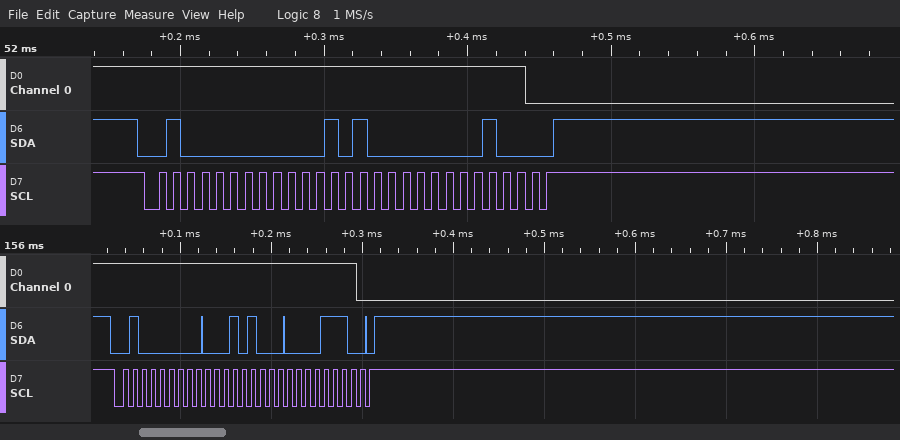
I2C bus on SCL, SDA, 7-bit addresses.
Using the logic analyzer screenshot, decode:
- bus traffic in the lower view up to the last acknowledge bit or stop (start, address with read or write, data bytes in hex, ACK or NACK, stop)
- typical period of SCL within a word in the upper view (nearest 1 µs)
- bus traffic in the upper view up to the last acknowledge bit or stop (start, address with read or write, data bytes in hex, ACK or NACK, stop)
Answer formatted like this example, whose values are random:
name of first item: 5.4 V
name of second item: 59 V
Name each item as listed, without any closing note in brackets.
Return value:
bus traffic in the lower view up to the last acknowledge bit or stop: start, address 20 write ACK, 14 ACK, 0E ACK, stop
typical period of SCL within a word in the upper view: 10 µs
bus traffic in the upper view up to the last acknowledge bit or stop: start, address 20 write ACK, 14 ACK, 04 ACK, stop
